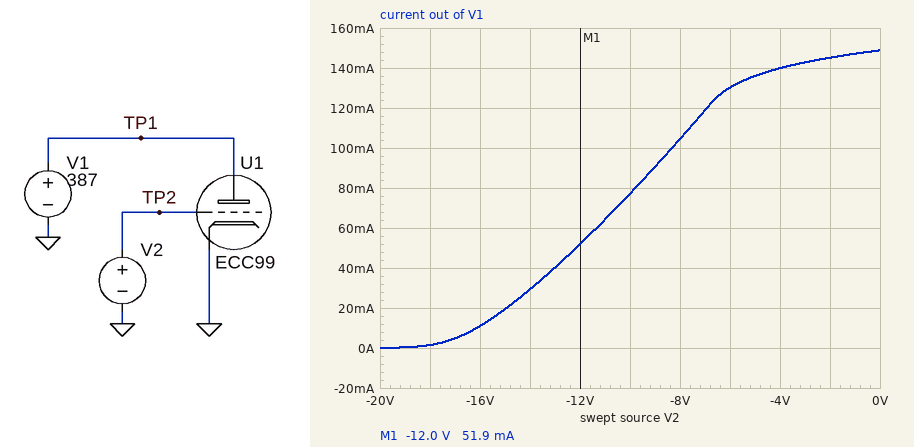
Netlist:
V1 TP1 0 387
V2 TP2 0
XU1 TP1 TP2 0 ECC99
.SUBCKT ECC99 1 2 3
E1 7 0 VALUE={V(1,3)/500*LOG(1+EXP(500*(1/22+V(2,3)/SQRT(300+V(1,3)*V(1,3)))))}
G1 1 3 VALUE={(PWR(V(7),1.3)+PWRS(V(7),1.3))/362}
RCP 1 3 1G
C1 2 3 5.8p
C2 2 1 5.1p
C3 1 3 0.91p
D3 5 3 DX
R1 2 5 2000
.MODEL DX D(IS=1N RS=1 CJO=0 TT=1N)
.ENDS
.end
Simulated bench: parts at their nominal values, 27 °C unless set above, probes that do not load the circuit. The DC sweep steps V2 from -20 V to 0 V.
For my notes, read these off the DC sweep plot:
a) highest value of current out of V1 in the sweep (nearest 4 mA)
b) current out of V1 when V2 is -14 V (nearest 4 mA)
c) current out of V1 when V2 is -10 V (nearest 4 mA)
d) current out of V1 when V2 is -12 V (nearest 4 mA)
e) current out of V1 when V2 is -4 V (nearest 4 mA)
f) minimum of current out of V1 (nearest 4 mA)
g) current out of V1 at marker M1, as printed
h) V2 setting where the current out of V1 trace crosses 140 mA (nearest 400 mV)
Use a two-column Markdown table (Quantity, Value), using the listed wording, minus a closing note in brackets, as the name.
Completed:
| Quantity | Value |
|---|---|
| highest value of current out of V1 in the sweep | 148 mA |
| current out of V1 when V2 is -14 V | 28 mA |
| current out of V1 when V2 is -10 V | 76 mA |
| current out of V1 when V2 is -12 V | 52 mA |
| current out of V1 when V2 is -4 V | 140 mA |
| minimum of current out of V1 | 0 A |
| current out of V1 at marker M1, as printed | 51.9 mA |
| V2 setting where the current out of V1 trace crosses 140 mA | -4.0 V |
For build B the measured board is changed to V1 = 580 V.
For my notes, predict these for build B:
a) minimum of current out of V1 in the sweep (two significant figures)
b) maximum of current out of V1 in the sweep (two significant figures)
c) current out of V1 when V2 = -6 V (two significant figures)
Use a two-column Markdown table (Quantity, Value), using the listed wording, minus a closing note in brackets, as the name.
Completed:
| Quantity | Value |
|---|---|
| minimum of current out of V1 in the sweep | 61 mA |
| maximum of current out of V1 in the sweep | 250 mA |
| current out of V1 when V2 = -6 V | 240 mA |
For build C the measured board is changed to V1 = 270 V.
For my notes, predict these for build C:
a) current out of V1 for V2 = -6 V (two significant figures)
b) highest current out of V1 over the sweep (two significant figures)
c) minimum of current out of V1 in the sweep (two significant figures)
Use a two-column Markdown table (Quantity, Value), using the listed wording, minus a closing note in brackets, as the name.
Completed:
| Quantity | Value |
|---|---|
| current out of V1 for V2 = -6 V | 60 mA |
| highest current out of V1 over the sweep | 93 mA |
| minimum of current out of V1 in the sweep | 270 nA |
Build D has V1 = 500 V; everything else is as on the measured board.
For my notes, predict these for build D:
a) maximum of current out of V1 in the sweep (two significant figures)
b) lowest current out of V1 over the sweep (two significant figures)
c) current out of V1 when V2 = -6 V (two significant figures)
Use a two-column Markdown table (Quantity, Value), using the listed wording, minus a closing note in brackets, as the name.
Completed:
| Quantity | Value |
|---|---|
| maximum of current out of V1 in the sweep | 210 mA |
| lowest current out of V1 over the sweep | 21 mA |
| current out of V1 when V2 = -6 V | 190 mA |
